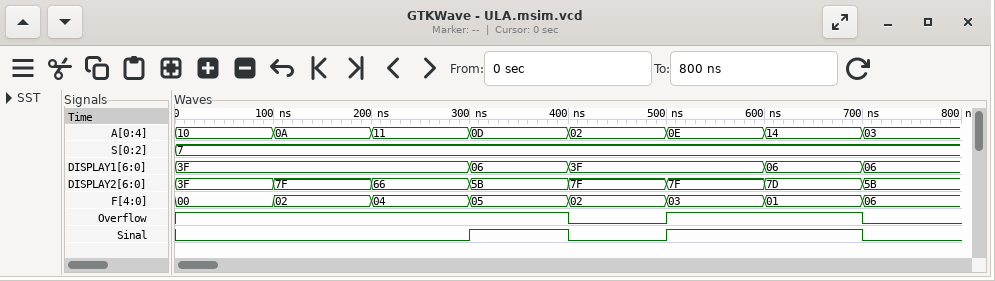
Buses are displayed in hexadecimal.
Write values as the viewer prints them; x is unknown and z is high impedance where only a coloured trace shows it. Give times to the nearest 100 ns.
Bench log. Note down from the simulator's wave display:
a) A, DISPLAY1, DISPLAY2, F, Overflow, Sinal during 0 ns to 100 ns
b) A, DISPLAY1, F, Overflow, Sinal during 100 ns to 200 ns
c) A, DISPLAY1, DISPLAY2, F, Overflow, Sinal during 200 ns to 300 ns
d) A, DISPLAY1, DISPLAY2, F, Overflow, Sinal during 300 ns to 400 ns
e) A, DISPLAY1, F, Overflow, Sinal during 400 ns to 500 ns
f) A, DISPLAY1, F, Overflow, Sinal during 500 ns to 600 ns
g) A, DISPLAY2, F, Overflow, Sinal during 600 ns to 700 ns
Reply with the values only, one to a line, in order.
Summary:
A=10, DISPLAY1=3F, DISPLAY2=3F, F=00, Overflow=1, Sinal=0
A=0A, DISPLAY1=3F, F=02, Overflow=1, Sinal=0
A=11, DISPLAY1=3F, DISPLAY2=66, F=04, Overflow=1, Sinal=0
A=0D, DISPLAY1=06, DISPLAY2=5B, F=05, Overflow=1, Sinal=1
A=02, DISPLAY1=3F, F=02, Overflow=0, Sinal=0
A=0E, DISPLAY1=3F, F=03, Overflow=1, Sinal=1
A=14, DISPLAY2=7D, F=01, Overflow=1, Sinal=1
